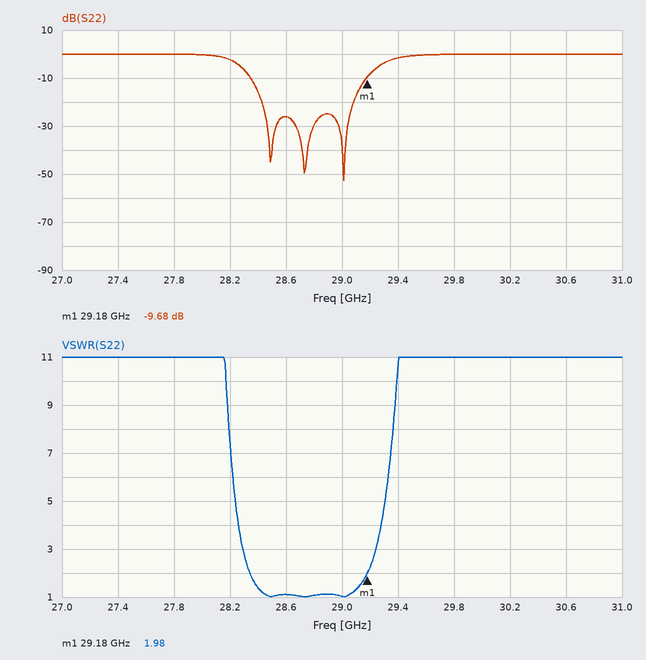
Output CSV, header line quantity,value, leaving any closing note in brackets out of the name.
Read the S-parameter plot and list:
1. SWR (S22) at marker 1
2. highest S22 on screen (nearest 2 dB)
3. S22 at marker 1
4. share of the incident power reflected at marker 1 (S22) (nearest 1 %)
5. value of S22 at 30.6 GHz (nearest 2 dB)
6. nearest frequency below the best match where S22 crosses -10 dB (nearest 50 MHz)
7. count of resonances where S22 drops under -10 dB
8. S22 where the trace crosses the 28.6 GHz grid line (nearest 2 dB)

quantity,value
SWR (S22) at marker 1,1.98
highest S22 on screen,0 dB
S22 at marker 1,-9.68 dB
share of the incident power reflected at marker 1 (S22),11 %
value of S22 at 30.6 GHz,0 dB
nearest frequency below the best match where S22 crosses -10 dB,28.35 GHz
count of resonances where S22 drops under -10 dB,3
S22 where the trace crosses the 28.6 GHz grid line,-26 dB
